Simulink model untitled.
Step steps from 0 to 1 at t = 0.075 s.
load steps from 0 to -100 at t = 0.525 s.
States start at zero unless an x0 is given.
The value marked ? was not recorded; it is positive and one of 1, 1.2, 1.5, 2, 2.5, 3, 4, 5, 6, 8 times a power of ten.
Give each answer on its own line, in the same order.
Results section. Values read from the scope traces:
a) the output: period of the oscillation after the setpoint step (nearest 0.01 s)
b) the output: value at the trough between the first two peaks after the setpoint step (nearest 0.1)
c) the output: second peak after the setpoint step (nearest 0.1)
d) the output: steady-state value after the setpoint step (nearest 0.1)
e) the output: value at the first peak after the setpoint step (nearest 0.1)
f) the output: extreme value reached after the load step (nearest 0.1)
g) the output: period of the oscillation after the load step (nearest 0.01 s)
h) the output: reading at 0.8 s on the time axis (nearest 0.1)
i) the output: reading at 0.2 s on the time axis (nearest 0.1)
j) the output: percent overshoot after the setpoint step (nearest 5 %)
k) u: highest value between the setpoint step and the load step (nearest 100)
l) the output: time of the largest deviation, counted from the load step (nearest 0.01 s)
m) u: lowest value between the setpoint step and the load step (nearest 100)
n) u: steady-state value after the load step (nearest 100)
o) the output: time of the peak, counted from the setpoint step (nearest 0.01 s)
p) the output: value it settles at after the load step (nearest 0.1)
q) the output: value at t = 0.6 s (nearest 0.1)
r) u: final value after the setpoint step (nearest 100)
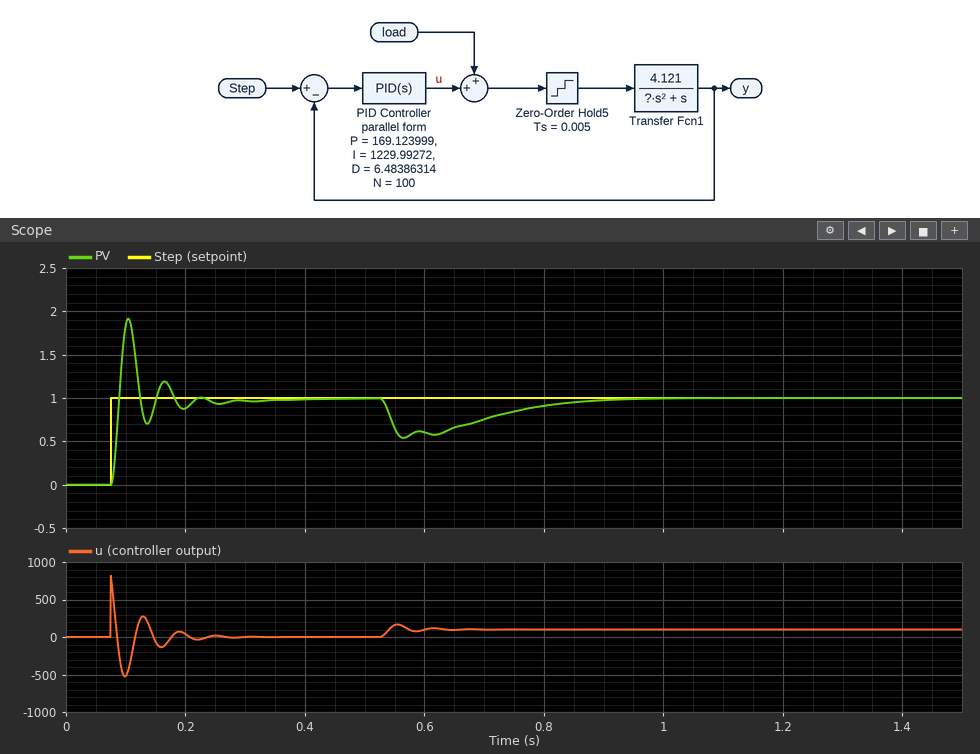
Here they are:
0.06 s
0.7
1.2
1.0
1.9
0.5
0.05 s
0.9
0.9
90 %
800
0.04 s
-500
100
0.03 s
1.0
0.6
0
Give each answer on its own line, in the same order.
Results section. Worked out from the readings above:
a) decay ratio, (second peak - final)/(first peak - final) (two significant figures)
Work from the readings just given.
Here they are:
0.22
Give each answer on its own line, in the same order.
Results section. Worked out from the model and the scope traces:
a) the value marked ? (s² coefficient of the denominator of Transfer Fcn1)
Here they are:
0.25
